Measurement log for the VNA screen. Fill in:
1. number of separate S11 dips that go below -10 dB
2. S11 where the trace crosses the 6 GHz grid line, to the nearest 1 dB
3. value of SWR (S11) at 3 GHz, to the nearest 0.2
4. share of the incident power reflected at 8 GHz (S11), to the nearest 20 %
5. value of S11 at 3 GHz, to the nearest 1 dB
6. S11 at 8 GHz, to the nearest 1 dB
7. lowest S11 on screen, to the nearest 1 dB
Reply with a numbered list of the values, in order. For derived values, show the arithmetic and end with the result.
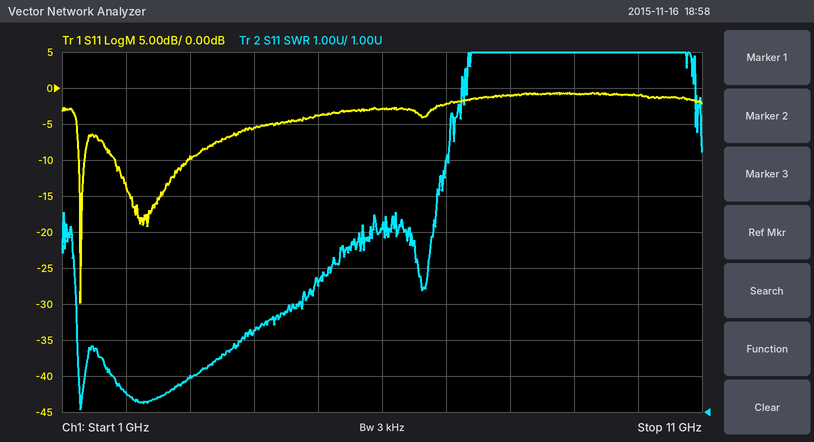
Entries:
1. 2
2. -3 dB
3. 2.0
4. 10^(-1/10) ≈ 79.4 %, so 80 % to the nearest 20 %
5. -10 dB
6. -1 dB
7. -30 dB
